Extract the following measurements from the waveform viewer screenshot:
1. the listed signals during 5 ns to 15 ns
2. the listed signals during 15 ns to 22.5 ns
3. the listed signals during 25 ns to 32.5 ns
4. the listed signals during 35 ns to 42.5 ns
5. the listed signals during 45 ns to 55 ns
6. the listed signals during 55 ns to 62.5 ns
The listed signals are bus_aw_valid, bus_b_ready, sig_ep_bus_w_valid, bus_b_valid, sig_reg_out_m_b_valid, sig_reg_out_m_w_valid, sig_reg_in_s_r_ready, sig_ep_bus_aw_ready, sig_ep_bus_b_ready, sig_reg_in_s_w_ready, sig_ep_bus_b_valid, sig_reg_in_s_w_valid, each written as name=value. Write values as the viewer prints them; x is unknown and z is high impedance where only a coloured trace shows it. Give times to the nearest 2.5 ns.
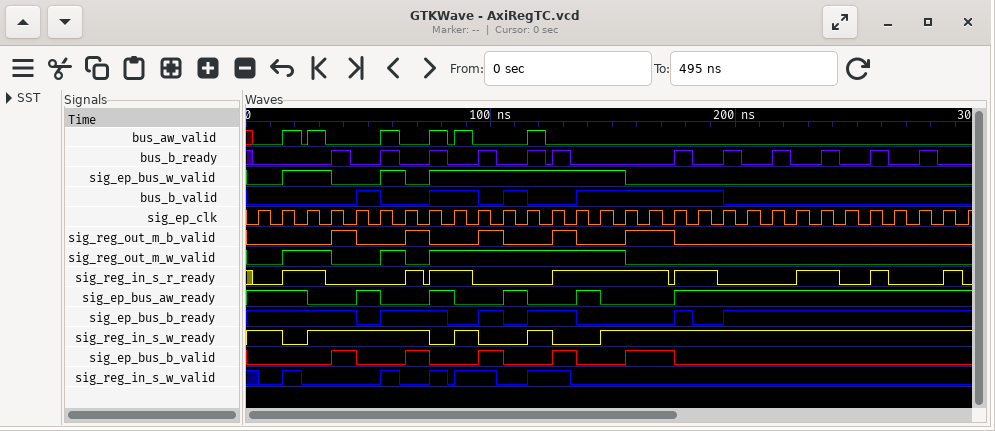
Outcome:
bus_aw_valid=0, bus_b_ready=0, sig_ep_bus_w_valid=0, bus_b_valid=0, sig_reg_out_m_b_valid=0, sig_reg_out_m_w_valid=0, sig_reg_in_s_r_ready=0, sig_ep_bus_aw_ready=1, sig_ep_bus_b_ready=1, sig_reg_in_s_w_ready=1, sig_ep_bus_b_valid=0, sig_reg_in_s_w_valid=0
bus_aw_valid=1, bus_b_ready=0, sig_ep_bus_w_valid=1, bus_b_valid=0, sig_reg_out_m_b_valid=0, sig_reg_out_m_w_valid=1, sig_reg_in_s_r_ready=1, sig_ep_bus_aw_ready=1, sig_ep_bus_b_ready=1, sig_reg_in_s_w_ready=0, sig_ep_bus_b_valid=0, sig_reg_in_s_w_valid=1
bus_aw_valid=1, bus_b_ready=0, sig_ep_bus_w_valid=1, bus_b_valid=0, sig_reg_out_m_b_valid=0, sig_reg_out_m_w_valid=1, sig_reg_in_s_r_ready=1, sig_ep_bus_aw_ready=0, sig_ep_bus_b_ready=1, sig_reg_in_s_w_ready=1, sig_ep_bus_b_valid=0, sig_reg_in_s_w_valid=0
bus_aw_valid=0, bus_b_ready=1, sig_ep_bus_w_valid=0, bus_b_valid=0, sig_reg_out_m_b_valid=1, sig_reg_out_m_w_valid=0, sig_reg_in_s_r_ready=0, sig_ep_bus_aw_ready=0, sig_ep_bus_b_ready=1, sig_reg_in_s_w_ready=1, sig_ep_bus_b_valid=1, sig_reg_in_s_w_valid=0
bus_aw_valid=0, bus_b_ready=0, sig_ep_bus_w_valid=0, bus_b_valid=1, sig_reg_out_m_b_valid=0, sig_reg_out_m_w_valid=0, sig_reg_in_s_r_ready=0, sig_ep_bus_aw_ready=1, sig_ep_bus_b_ready=0, sig_reg_in_s_w_ready=1, sig_ep_bus_b_valid=0, sig_reg_in_s_w_valid=0
bus_aw_valid=1, bus_b_ready=1, sig_ep_bus_w_valid=1, bus_b_valid=0, sig_reg_out_m_b_valid=0, sig_reg_out_m_w_valid=1, sig_reg_in_s_r_ready=0, sig_ep_bus_aw_ready=0, sig_ep_bus_b_ready=1, sig_reg_in_s_w_ready=1, sig_ep_bus_b_valid=0, sig_reg_in_s_w_valid=1
